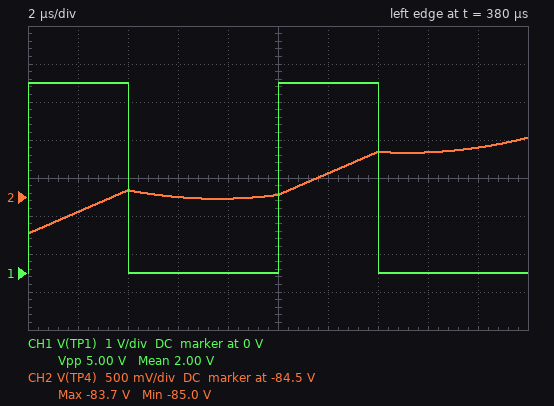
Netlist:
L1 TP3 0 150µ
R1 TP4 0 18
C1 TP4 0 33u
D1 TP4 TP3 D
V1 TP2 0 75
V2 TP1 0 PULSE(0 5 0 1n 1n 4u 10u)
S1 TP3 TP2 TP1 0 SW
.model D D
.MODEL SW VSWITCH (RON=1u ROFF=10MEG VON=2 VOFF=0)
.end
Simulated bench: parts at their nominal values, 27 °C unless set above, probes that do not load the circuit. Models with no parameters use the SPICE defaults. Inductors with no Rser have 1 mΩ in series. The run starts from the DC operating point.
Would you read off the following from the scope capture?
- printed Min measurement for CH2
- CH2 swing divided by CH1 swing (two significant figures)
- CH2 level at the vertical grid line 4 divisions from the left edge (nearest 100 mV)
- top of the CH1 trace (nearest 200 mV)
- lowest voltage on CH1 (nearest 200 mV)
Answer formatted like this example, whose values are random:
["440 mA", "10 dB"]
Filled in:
["-85.0 V", "0.25", "-84.5 V", "5.0 V", "0 V"]
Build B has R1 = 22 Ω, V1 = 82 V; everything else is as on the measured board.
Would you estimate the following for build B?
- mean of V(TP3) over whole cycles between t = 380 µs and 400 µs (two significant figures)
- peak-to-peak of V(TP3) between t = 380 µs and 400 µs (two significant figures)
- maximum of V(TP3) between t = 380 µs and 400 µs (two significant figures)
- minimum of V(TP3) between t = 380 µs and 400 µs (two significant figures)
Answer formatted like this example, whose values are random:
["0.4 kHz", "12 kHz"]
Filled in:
["-24 V", "180 V", "82 V", "-96 V"]
